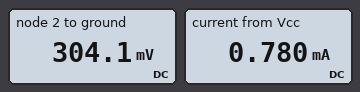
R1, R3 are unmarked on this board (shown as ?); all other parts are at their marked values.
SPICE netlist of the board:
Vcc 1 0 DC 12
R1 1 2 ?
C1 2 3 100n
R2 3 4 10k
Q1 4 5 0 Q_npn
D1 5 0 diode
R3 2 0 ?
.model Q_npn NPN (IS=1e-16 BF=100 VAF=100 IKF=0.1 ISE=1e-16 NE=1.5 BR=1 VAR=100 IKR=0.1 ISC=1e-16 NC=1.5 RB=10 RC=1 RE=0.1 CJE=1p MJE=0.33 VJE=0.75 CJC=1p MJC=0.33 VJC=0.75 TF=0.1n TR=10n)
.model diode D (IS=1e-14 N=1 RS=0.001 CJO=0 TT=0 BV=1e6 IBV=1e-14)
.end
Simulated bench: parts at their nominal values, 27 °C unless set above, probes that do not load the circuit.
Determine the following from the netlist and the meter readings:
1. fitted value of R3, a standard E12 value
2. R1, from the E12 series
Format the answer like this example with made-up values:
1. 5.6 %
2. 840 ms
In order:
1. 390 Ω
2. 15 kΩ
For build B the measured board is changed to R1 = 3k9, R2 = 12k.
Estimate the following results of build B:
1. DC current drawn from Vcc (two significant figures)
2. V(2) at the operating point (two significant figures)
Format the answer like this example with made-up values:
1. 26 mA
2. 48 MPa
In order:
1. 2.8 mA
2. 1.1 V
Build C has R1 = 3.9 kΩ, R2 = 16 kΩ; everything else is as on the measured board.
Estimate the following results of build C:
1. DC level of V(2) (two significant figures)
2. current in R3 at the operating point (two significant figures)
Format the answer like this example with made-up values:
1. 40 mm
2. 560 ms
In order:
1. 1.1 V
2. 2.8 mA
